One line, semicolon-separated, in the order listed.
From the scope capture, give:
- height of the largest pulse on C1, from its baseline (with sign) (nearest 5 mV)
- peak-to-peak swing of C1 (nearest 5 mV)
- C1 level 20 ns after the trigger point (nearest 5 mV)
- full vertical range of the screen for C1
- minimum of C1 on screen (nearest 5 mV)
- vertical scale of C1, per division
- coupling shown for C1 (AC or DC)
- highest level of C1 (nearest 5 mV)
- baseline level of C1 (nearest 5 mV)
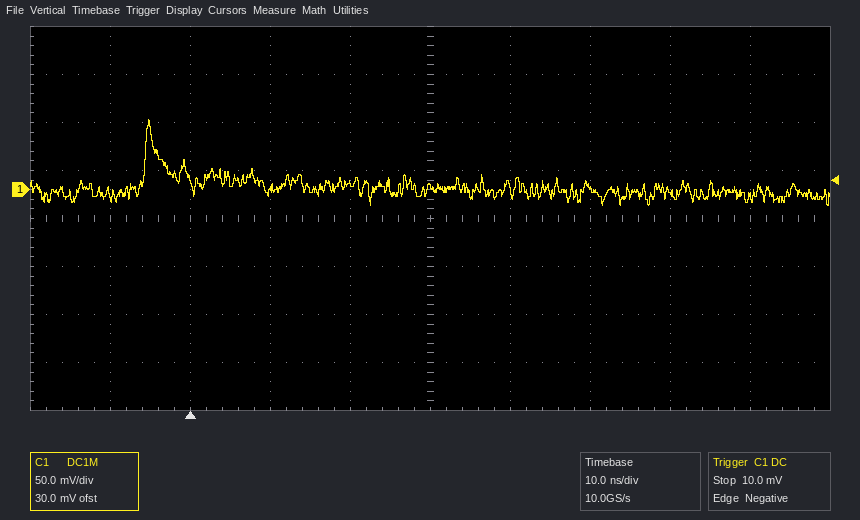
+75 mV; 90 mV; 5 mV; 400 mV; -15 mV; 50 mV; DC; 75 mV; 0 mV
